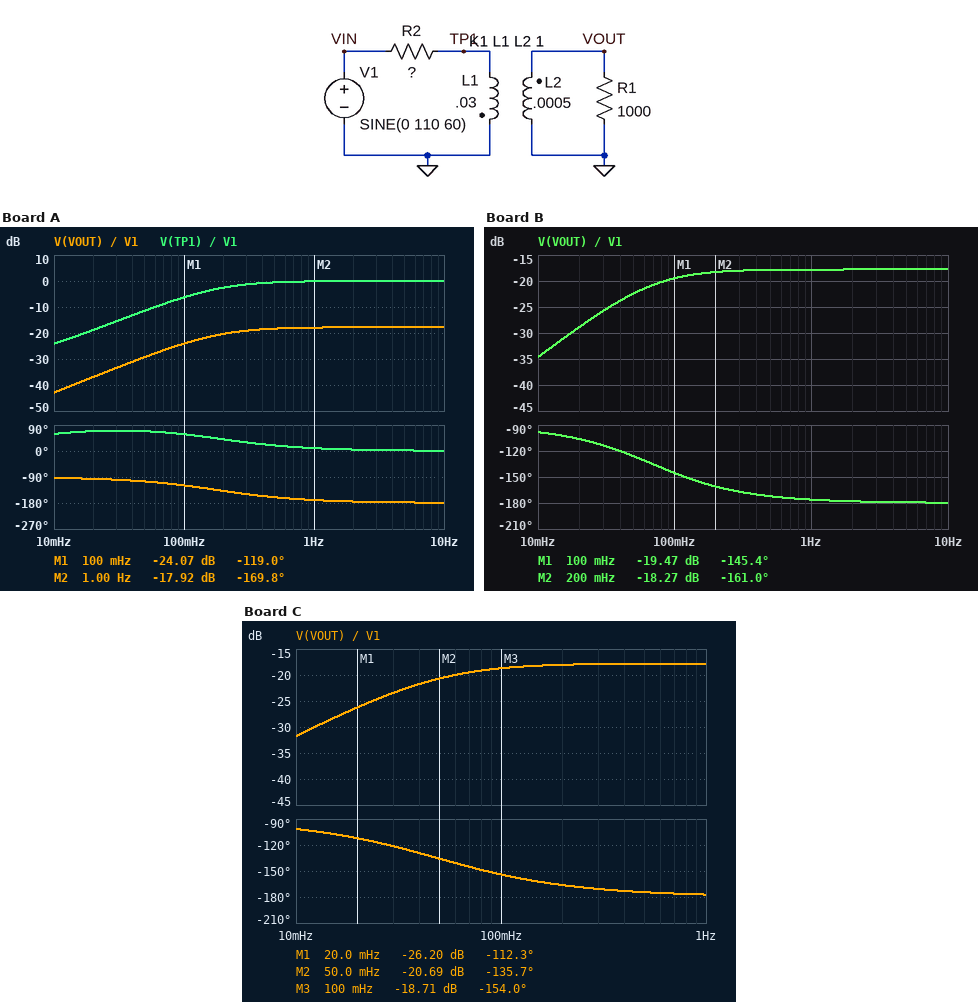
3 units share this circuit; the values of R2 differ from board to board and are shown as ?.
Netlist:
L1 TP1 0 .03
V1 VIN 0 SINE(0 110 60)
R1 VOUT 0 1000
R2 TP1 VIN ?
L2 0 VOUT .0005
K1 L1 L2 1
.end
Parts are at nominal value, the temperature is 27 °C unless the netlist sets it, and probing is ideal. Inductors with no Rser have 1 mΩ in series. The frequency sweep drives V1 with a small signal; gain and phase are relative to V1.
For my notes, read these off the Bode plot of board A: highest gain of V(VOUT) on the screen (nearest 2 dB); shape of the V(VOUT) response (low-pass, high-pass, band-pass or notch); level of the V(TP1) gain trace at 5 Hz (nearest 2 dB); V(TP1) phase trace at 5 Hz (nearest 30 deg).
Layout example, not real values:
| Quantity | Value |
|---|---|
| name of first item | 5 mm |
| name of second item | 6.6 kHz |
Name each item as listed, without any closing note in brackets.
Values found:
| Quantity | Value |
|---|---|
| highest gain of V(VOUT) on the screen | -18 dB |
| shape of the V(VOUT) response | high-pass |
| level of the V(TP1) gain trace at 5 Hz | 0 dB |
| V(TP1) phase trace at 5 Hz | 0 deg |
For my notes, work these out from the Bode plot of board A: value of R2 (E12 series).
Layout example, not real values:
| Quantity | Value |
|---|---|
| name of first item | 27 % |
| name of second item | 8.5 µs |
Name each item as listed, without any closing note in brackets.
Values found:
| Quantity | Value |
|---|---|
| value of R2 | 0.033 Ω |
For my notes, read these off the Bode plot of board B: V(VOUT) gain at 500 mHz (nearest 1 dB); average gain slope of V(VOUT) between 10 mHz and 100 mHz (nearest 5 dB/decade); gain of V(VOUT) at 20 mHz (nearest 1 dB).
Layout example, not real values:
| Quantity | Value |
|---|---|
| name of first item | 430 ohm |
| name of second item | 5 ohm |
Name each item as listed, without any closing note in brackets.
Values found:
| Quantity | Value |
|---|---|
| V(VOUT) gain at 500 mHz | -18 dB |
| average gain slope of V(VOUT) between 10 mHz and 100 mHz | 15 dB/decade |
| gain of V(VOUT) at 20 mHz | -29 dB |
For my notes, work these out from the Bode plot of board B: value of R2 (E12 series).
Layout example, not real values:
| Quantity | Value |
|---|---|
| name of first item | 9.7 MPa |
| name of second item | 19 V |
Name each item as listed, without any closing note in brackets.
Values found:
| Quantity | Value |
|---|---|
| value of R2 | 0.012 Ω |
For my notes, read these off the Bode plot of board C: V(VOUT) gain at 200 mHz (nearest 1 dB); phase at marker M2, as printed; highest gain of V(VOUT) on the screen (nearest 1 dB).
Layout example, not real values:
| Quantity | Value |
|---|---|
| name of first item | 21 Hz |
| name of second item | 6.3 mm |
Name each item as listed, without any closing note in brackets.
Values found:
| Quantity | Value |
|---|---|
| V(VOUT) gain at 200 mHz | -18 dB |
| phase at marker M2, as printed | -135.7 deg |
| highest gain of V(VOUT) on the screen | -18 dB |
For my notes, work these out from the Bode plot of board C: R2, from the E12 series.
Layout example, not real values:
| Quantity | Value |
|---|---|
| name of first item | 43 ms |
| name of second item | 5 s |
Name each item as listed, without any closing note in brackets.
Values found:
| Quantity | Value |
|---|---|
| R2, from the E12 series | 8.2 mΩ |
